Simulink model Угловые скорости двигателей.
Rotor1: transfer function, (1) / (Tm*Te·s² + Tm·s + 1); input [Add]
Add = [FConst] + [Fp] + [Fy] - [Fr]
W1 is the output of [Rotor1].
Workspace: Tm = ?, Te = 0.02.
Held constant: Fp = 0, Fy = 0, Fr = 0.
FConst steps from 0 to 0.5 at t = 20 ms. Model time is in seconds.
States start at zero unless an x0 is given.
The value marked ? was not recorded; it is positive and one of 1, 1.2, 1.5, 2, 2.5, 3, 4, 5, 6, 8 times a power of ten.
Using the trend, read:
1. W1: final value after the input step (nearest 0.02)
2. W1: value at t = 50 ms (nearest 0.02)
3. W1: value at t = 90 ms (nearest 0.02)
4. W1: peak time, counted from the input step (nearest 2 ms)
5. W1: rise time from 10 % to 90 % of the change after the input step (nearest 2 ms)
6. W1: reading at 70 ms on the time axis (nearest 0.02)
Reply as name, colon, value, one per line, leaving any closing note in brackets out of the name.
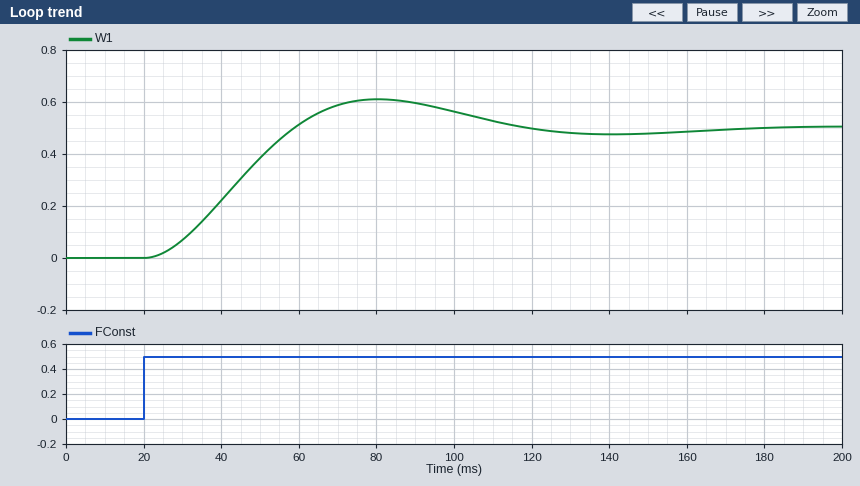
W1: final value after the input step: 0.50
W1: value at t = 50 ms: 0.38
W1: value at t = 90 ms: 0.60
W1: peak time, counted from the input step: 60 ms
W1: rise time from 10 % to 90 % of the change after the input step: 26 ms
W1: reading at 70 ms on the time axis: 0.58
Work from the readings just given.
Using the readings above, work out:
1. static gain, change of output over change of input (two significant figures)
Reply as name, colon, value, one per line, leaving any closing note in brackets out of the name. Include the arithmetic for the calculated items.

static gain, change of output over change of input: (0.5 - 0) / (0.5 - 0) = 1.0
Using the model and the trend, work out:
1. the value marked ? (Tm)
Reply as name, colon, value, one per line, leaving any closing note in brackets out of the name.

the value marked ?: 0.015
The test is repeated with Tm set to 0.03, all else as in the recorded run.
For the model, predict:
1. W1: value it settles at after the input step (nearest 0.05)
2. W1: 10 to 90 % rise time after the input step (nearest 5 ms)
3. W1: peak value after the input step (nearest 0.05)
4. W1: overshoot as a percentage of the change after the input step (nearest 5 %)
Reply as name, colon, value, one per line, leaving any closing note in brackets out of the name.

W1: value it settles at after the input step: 0.50
W1: 10 to 90 % rise time after the input step: 45 ms
W1: peak value after the input step: 0.55
W1: overshoot as a percentage of the change after the input step: 10 %
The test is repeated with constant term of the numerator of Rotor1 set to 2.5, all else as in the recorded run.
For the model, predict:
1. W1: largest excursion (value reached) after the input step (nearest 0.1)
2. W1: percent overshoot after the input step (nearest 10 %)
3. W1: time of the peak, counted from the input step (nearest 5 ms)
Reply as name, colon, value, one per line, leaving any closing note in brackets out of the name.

W1: largest excursion (value reached) after the input step: 1.5
W1: percent overshoot after the input step: 20 %
W1: time of the peak, counted from the input step: 60 ms
